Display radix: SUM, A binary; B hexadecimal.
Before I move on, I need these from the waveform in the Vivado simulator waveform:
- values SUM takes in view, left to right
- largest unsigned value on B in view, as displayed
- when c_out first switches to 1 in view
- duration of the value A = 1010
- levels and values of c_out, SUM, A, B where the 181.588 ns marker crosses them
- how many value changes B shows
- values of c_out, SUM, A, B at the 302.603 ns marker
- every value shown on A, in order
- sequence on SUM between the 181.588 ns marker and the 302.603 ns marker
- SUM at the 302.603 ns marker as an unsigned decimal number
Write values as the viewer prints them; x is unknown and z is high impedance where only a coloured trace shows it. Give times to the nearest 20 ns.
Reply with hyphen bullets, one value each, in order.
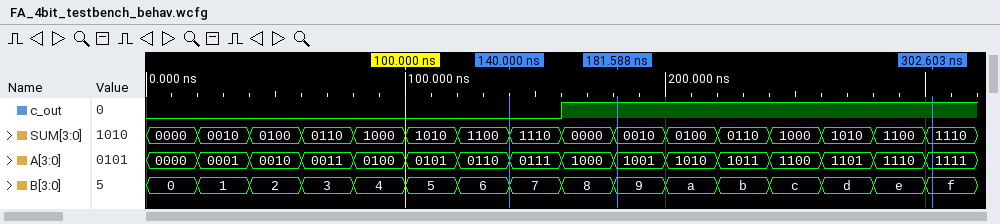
- 0000, 0010, 0100, 0110, 1000, 1010, 1100, 1110, 0000, 0010, 0100, 0110, 1000, 1010, 1100, 1110
- f
- 160 ns
- 20 ns
- c_out=1, SUM=0010, A=1001, B=9
- 15
- c_out=1, SUM=1110, A=1111, B=f
- 0000, 0001, 0010, 0011, 0100, 0101, 0110, 0111, 1000, 1001, 1010, 1011, 1100, 1101, 1110, 1111
- 0010, 0100, 0110, 1000, 1010, 1100, 1110
- 14
